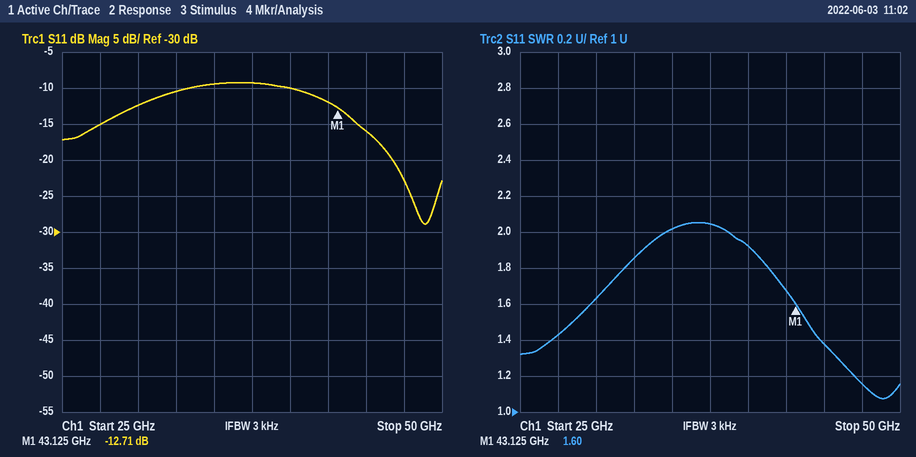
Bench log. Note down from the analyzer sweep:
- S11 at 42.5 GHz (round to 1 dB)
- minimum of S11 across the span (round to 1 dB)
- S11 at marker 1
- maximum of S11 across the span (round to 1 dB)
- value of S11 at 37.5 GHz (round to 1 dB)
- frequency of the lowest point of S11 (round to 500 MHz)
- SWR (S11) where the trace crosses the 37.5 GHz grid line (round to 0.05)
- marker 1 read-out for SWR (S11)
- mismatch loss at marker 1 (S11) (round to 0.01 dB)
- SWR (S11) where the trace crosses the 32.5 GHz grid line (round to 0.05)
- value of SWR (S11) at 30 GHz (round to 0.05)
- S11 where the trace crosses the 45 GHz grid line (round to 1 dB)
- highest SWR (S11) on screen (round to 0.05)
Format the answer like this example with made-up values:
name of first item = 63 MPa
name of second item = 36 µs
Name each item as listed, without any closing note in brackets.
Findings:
S11 at 42.5 GHz = -12 dB
minimum of S11 across the span = -29 dB
S11 at marker 1 = -12.71 dB
maximum of S11 across the span = -9 dB
value of S11 at 37.5 GHz = -9 dB
frequency of the lowest point of S11 = 49.0 GHz
SWR (S11) where the trace crosses the 37.5 GHz grid line = 2.05
marker 1 read-out for SWR = 1.60
mismatch loss at marker 1 (S11) = 0.24 dB
SWR (S11) where the trace crosses the 32.5 GHz grid line = 1.85
value of SWR (S11) at 30 GHz = 1.65
S11 where the trace crosses the 45 GHz grid line = -16 dB
highest SWR (S11) on screen = 2.05
